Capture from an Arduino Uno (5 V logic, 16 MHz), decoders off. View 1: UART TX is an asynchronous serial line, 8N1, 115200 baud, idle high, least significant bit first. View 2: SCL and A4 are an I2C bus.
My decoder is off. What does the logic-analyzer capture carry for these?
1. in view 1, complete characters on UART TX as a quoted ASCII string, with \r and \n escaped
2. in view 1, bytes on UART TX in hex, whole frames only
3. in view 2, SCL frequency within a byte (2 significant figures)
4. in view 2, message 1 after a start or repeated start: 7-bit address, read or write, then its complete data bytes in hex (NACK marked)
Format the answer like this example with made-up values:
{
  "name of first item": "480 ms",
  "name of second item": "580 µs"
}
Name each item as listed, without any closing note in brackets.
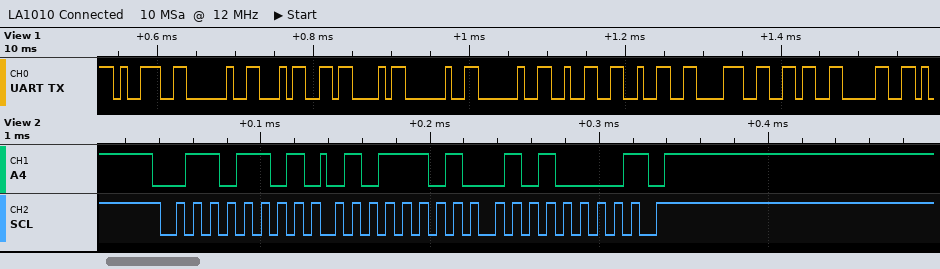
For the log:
{
  "in view 1, complete characters on UART TX as a quoted ASCII string, with \\r and \\n escaped": "\"9 4C  22860\"",
  "in view 1, bytes on UART TX in hex, whole frames only": "39 20 34 43 20 20 32 32 38 36 30",
  "in view 2, SCL frequency within a byte": "100 kHz",
  "in view 2, message 1 after a start or repeated start: 7-bit address, read or write, then its complete data bytes in hex": "0x36 read: 5D 50 NACK"
}
